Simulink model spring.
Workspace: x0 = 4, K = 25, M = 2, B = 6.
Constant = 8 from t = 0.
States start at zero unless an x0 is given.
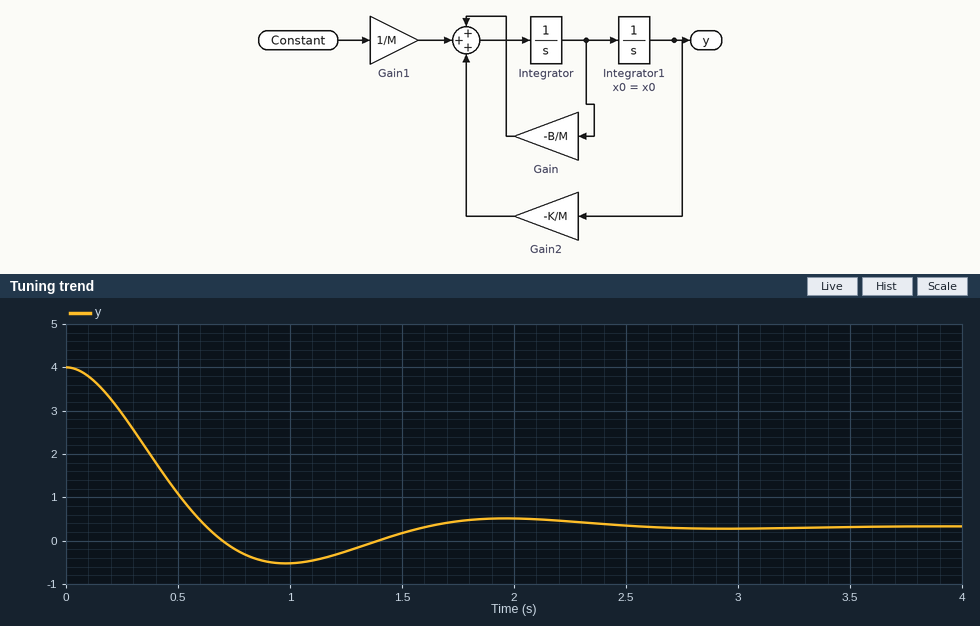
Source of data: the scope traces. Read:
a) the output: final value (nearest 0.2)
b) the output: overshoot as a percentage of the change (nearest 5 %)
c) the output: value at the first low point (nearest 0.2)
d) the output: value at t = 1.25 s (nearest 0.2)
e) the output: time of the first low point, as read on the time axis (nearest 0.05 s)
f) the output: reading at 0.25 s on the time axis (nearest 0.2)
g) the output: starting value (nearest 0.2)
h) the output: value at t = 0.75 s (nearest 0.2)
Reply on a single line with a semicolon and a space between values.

0.4; 25 %; -0.6; -0.2; 1.00 s; 3.0; 4.0; -0.2
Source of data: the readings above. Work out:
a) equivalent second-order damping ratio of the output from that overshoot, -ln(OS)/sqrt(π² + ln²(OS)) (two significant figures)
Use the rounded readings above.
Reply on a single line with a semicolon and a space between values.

0.40
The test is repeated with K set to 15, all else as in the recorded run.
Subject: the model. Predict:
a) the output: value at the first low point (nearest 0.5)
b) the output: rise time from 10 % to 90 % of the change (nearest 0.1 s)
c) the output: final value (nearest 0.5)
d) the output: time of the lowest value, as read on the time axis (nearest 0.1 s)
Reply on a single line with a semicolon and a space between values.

0.0; 0.6 s; 0.5; 1.4 s
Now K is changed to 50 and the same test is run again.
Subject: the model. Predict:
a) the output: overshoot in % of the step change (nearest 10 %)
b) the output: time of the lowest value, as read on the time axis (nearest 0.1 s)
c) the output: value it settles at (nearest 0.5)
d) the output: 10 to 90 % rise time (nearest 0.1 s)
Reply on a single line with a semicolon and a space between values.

40 %; 0.7 s; 0.0; 0.3 s
